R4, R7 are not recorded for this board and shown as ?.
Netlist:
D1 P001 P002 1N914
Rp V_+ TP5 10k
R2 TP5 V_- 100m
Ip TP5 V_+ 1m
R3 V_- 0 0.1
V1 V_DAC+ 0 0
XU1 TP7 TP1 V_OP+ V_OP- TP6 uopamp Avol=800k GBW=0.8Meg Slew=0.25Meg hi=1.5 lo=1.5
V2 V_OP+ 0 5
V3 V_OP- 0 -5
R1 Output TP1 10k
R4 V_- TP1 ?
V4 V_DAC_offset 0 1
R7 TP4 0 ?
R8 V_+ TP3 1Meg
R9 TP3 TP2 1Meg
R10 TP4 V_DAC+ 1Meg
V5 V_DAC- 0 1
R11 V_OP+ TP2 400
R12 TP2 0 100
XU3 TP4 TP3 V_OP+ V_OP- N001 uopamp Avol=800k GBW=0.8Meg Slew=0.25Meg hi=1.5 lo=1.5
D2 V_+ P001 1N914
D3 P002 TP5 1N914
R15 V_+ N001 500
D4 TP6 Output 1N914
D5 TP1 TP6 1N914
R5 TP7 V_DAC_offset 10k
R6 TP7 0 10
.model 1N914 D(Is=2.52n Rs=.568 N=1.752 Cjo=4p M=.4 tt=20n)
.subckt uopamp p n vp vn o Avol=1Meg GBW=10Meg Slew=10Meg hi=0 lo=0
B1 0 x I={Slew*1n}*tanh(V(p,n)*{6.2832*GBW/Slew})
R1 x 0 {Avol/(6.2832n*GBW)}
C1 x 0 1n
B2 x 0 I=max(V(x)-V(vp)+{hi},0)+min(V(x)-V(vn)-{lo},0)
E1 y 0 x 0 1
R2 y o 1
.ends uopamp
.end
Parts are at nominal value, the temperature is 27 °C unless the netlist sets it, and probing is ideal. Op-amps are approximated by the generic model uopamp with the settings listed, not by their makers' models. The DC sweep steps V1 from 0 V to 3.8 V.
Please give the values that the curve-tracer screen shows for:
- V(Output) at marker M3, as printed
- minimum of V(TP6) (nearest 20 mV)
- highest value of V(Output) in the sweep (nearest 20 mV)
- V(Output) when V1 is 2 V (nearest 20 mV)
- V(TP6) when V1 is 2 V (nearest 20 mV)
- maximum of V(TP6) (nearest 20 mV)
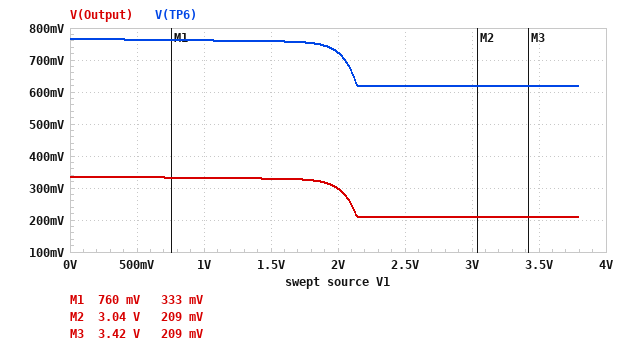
209 mV
620 mV
340 mV
300 mV
720 mV
760 mV
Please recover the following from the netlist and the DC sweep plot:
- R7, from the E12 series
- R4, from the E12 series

2.2 MΩ
33 Ω
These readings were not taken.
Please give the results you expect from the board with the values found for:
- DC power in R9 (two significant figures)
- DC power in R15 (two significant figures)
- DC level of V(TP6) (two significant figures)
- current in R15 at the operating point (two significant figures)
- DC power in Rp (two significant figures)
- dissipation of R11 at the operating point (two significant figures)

1.0 µW
610 µW
770 mV
1.1 mA
100 µW
40 mW
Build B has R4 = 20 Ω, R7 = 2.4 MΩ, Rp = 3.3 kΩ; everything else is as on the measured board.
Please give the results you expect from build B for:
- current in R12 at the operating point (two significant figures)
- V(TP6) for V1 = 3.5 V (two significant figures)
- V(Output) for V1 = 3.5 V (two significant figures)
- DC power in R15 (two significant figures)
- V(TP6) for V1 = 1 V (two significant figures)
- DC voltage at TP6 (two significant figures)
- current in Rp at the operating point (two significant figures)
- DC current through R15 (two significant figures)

10 mA
770 mV
340 mV
850 µW
990 mV
1.0 V
300 µA
1.3 mA
